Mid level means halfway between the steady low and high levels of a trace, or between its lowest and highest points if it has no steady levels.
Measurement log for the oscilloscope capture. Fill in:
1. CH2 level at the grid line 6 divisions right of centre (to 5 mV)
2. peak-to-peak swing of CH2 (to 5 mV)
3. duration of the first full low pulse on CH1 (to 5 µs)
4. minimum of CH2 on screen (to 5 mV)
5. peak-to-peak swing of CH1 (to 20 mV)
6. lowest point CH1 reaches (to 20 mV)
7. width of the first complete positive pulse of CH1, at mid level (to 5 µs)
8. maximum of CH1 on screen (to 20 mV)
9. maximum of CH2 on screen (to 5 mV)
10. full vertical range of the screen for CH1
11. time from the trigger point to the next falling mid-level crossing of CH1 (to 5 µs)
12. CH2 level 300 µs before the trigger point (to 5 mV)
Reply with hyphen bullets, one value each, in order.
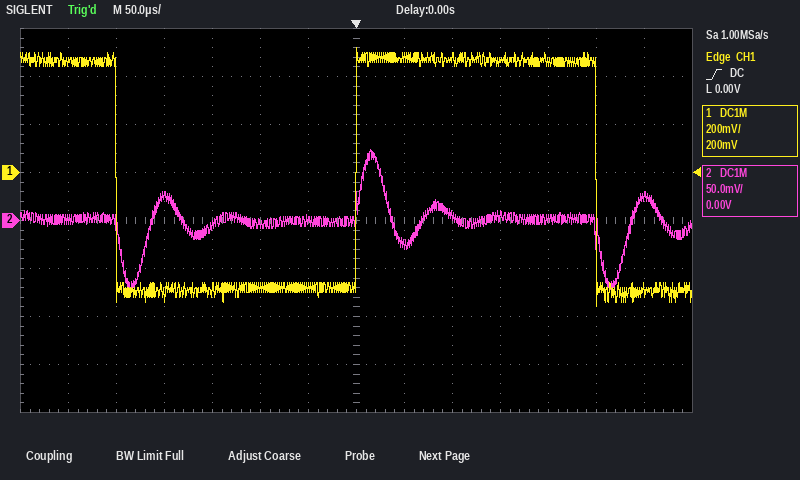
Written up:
- 25 mV
- 145 mV
- 250 µs
- -70 mV
- 1.08 V
- -560 mV
- 250 µs
- 520 mV
- 75 mV
- 1.6 V
- 250 µs
- 0 mV
